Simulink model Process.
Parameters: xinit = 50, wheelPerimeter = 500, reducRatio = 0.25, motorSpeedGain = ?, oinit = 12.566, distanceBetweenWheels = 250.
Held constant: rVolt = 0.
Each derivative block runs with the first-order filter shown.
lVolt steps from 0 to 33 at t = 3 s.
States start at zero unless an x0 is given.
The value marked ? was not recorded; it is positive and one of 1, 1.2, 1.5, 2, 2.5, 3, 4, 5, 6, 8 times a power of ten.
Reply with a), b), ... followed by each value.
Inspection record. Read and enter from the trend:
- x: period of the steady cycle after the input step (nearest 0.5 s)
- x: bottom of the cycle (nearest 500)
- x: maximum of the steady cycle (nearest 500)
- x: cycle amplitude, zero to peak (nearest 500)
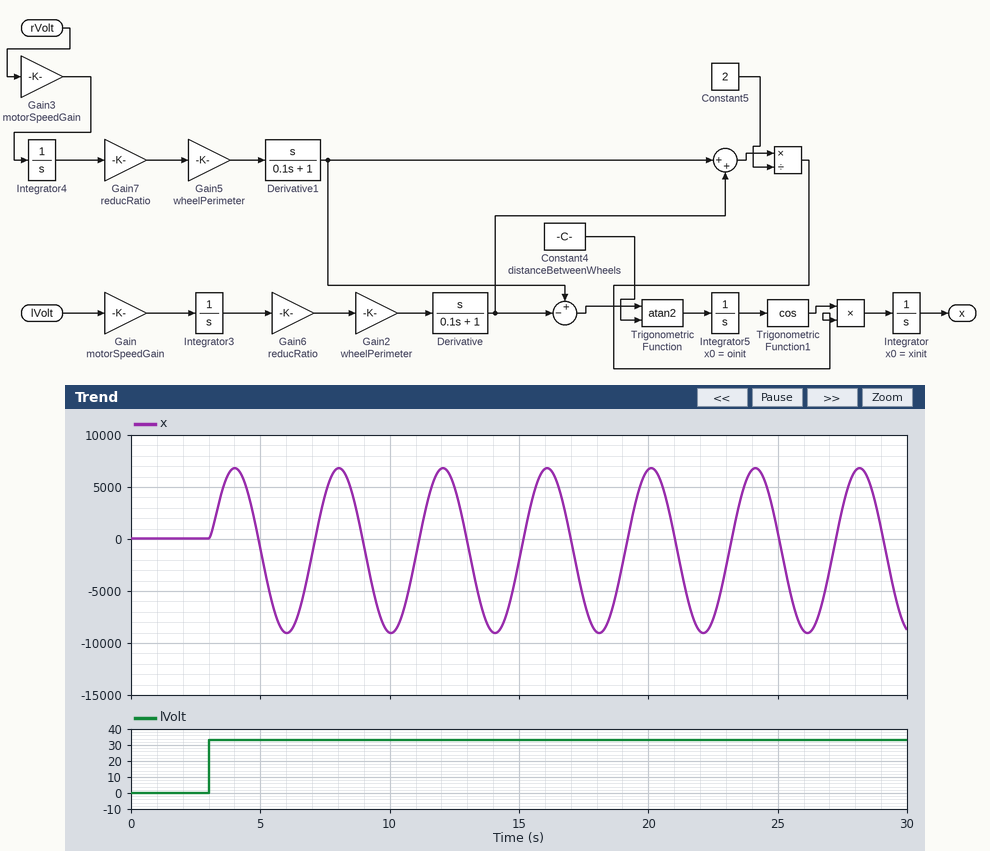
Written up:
a) 4.0 s
b) -9000
c) 7000
d) 8000
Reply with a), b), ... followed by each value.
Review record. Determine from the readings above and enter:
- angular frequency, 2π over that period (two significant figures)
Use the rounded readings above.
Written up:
a) 1.6 rad/s
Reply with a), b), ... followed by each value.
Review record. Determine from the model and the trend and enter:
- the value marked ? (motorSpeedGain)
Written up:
a) 6
